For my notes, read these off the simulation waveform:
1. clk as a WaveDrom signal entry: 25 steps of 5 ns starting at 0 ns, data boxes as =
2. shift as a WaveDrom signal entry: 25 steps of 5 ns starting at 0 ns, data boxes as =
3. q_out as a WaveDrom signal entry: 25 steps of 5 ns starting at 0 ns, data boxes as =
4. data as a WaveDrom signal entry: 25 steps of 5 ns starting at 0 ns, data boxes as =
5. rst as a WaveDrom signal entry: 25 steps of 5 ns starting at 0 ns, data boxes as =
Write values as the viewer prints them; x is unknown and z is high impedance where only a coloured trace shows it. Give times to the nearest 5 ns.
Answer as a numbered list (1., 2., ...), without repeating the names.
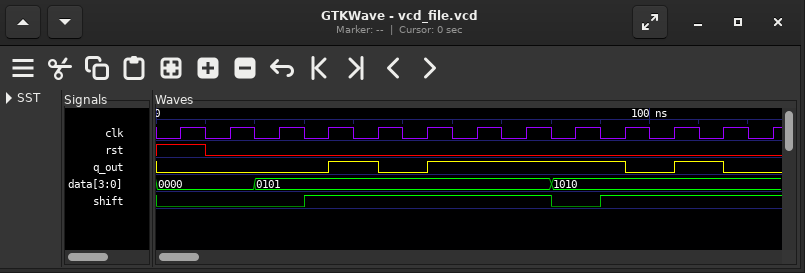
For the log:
1. {name: 'clk', wave: '0101010101010101010101010'}
2. {name: 'shift', wave: '0.....1.........0.1......'}
3. {name: 'q_out', wave: '0......1.0.1.......0.1.0.'}
4. {name: 'data', wave: '=...=...........=........', data: '0000 0101 1010'}
5. {name: 'rst', wave: '1.0......................'}
